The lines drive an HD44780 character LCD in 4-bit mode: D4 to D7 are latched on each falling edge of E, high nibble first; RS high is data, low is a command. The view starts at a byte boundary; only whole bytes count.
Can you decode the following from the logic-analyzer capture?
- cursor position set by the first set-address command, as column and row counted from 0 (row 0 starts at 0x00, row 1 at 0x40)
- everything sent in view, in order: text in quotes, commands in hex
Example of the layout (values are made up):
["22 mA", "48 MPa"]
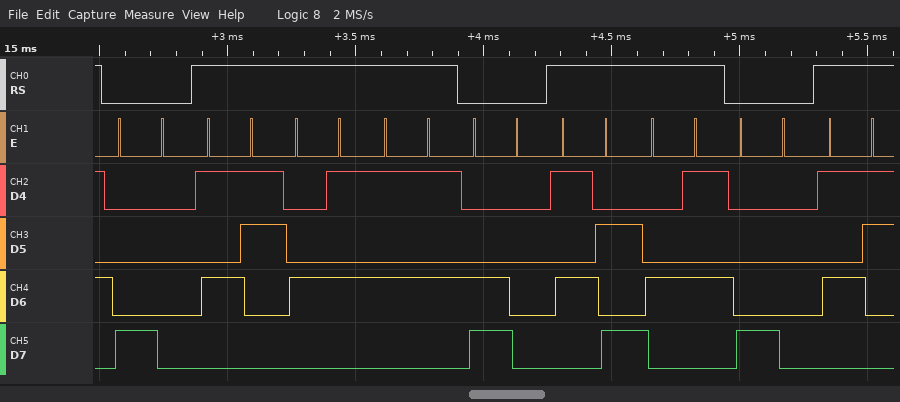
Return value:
["column 0, row 0", "0x80 \"SEU\" 0xC0 \"ZE\" 0x80 \"S\""]
